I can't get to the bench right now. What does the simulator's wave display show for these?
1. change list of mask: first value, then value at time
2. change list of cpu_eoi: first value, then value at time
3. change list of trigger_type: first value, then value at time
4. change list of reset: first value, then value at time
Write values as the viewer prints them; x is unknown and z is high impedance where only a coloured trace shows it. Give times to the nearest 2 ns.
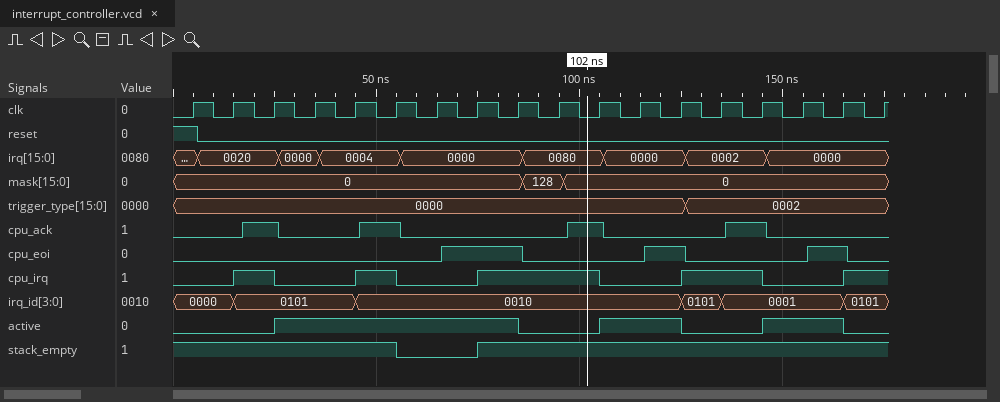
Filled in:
0, 128 at 86 ns, 0 at 96 ns
0, 1 at 66 ns, 0 at 86 ns, 1 at 116 ns, 0 at 126 ns, 1 at 156 ns, 0 at 166 ns
0000, 0002 at 126 ns
1, 0 at 6 ns
